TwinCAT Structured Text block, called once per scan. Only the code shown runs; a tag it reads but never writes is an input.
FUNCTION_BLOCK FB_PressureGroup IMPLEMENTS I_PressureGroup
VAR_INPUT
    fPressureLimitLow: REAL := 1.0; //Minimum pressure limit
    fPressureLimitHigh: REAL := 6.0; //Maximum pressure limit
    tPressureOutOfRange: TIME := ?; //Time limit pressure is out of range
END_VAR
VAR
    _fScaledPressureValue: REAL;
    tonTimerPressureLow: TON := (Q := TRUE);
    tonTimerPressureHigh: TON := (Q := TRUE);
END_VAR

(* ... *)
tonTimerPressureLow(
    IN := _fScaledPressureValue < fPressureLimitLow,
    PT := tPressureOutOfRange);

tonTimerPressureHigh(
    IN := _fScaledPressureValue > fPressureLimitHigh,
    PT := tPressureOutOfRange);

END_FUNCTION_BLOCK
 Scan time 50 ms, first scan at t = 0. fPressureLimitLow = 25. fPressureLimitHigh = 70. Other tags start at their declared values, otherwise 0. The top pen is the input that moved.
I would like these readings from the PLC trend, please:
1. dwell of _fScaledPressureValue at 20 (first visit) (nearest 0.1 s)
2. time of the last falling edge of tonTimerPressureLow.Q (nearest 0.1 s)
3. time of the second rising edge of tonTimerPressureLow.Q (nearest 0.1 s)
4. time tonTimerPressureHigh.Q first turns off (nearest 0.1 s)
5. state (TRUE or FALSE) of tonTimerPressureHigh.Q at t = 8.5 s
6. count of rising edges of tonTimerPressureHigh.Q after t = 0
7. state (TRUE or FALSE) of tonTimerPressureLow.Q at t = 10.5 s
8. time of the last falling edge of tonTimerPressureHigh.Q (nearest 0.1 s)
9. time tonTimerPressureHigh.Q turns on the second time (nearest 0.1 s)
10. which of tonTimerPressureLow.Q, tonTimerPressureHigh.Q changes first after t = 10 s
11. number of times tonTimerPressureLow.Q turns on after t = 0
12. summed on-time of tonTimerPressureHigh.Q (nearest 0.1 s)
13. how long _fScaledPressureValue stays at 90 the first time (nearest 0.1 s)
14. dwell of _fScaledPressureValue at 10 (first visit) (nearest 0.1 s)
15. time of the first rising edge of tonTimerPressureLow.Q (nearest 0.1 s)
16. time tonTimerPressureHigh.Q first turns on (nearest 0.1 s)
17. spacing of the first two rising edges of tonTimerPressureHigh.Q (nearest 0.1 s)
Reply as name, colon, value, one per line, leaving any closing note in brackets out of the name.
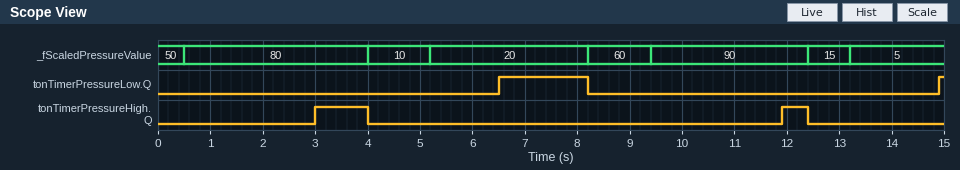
dwell of _fScaledPressureValue at 20 (first visit): 3.0 s
time of the last falling edge of tonTimerPressureLow.Q: 8.2 s
time of the second rising edge of tonTimerPressureLow.Q: 14.9 s
time tonTimerPressureHigh.Q first turns off: 4.0 s
state (TRUE or FALSE) of tonTimerPressureHigh.Q at t = 8.5 s: FALSE
count of rising edges of tonTimerPressureHigh.Q after t = 0: 2
state (TRUE or FALSE) of tonTimerPressureLow.Q at t = 10.5 s: FALSE
time of the last falling edge of tonTimerPressureHigh.Q: 12.4 s
time tonTimerPressureHigh.Q turns on the second time: 11.9 s
which of tonTimerPressureLow.Q, tonTimerPressureHigh.Q changes first after t = 10 s: tonTimerPressureHigh.Q
number of times tonTimerPressureLow.Q turns on after t = 0: 2
summed on-time of tonTimerPressureHigh.Q: 1.5 s
how long _fScaledPressureValue stays at 90 the first time: 3.0 s
dwell of _fScaledPressureValue at 10 (first visit): 1.2 s
time of the first rising edge of tonTimerPressureLow.Q: 6.5 s
time tonTimerPressureHigh.Q first turns on: 3.0 s
spacing of the first two rising edges of tonTimerPressureHigh.Q: 8.9 s
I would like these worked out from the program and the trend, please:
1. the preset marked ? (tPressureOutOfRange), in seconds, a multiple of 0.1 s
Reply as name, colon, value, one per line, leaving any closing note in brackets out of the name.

the preset marked ? (tPressureOutOfRange), in seconds, a multiple of 0.1 s: 2.5 s
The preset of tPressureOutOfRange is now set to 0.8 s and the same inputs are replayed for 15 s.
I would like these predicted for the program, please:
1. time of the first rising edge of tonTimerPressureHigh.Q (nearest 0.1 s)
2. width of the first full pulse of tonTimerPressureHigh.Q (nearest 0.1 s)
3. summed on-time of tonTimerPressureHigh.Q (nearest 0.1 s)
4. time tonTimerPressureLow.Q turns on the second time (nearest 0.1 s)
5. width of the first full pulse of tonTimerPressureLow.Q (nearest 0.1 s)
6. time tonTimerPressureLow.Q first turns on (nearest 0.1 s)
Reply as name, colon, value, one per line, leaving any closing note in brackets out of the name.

time of the first rising edge of tonTimerPressureHigh.Q: 1.3 s
width of the first full pulse of tonTimerPressureHigh.Q: 2.7 s
summed on-time of tonTimerPressureHigh.Q: 4.9 s
time tonTimerPressureLow.Q turns on the second time: 13.2 s
width of the first full pulse of tonTimerPressureLow.Q: 3.4 s
time tonTimerPressureLow.Q first turns on: 4.8 s
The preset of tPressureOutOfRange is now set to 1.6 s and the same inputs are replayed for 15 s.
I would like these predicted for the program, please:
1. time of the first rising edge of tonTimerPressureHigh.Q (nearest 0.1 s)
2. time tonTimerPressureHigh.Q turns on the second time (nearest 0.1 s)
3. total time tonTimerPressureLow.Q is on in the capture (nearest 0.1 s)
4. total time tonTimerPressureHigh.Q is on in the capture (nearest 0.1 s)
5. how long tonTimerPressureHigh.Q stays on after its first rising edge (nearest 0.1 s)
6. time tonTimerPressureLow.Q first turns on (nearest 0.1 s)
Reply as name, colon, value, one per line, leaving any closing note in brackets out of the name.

time of the first rising edge of tonTimerPressureHigh.Q: 2.1 s
time tonTimerPressureHigh.Q turns on the second time: 11.0 s
total time tonTimerPressureLow.Q is on in the capture: 3.6 s
total time tonTimerPressureHigh.Q is on in the capture: 3.3 s
how long tonTimerPressureHigh.Q stays on after its first rising edge: 1.9 s
time tonTimerPressureLow.Q first turns on: 5.6 s
